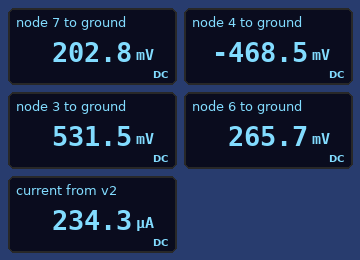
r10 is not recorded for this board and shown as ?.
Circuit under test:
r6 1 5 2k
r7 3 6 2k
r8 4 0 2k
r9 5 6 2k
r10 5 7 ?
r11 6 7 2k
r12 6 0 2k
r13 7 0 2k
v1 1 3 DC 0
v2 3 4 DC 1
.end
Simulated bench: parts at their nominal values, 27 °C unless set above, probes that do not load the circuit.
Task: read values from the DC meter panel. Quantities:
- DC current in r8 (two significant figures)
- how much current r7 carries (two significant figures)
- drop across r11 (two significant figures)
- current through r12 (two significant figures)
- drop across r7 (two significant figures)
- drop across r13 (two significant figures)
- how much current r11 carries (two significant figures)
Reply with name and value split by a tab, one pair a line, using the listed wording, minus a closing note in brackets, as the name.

DC current in r8	230 µA
how much current r7 carries	130 µA
drop across r11	63 mV
current through r12	130 µA
drop across r7	270 mV
drop across r13	200 mV
how much current r11 carries	31 µA
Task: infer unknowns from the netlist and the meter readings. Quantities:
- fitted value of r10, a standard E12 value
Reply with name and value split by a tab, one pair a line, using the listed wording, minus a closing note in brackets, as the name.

fitted value of r10, a standard E12 value	1.8 kΩ
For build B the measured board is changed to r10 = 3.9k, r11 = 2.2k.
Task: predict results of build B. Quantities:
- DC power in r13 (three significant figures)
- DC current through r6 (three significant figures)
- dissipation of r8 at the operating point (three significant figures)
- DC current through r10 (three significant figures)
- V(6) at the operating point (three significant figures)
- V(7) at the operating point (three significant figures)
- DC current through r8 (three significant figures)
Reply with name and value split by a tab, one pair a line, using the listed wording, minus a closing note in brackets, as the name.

DC power in r13	16.2 µW
DC current through r6	91.4 µA
dissipation of r8 at the operating point	103 µW
DC current through r10	47.0 µA
V(6) at the operating point	274 mV
V(7) at the operating point	180 mV
DC current through r8	227 µA
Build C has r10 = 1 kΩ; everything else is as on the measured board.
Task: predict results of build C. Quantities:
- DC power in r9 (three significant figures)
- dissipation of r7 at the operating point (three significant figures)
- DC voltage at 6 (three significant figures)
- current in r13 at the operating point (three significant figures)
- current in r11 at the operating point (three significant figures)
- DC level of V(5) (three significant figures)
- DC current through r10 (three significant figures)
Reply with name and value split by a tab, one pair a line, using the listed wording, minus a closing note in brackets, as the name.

DC power in r9	945 nW
dissipation of r7 at the operating point	34.0 µW
DC voltage at 6	261 mV
current in r13 at the operating point	109 µA
current in r11 at the operating point	21.7 µA
DC level of V(5)	304 mV
DC current through r10	87.0 µA
